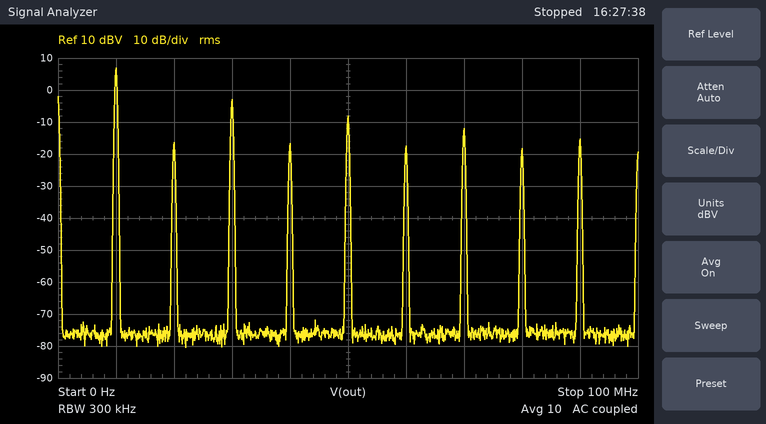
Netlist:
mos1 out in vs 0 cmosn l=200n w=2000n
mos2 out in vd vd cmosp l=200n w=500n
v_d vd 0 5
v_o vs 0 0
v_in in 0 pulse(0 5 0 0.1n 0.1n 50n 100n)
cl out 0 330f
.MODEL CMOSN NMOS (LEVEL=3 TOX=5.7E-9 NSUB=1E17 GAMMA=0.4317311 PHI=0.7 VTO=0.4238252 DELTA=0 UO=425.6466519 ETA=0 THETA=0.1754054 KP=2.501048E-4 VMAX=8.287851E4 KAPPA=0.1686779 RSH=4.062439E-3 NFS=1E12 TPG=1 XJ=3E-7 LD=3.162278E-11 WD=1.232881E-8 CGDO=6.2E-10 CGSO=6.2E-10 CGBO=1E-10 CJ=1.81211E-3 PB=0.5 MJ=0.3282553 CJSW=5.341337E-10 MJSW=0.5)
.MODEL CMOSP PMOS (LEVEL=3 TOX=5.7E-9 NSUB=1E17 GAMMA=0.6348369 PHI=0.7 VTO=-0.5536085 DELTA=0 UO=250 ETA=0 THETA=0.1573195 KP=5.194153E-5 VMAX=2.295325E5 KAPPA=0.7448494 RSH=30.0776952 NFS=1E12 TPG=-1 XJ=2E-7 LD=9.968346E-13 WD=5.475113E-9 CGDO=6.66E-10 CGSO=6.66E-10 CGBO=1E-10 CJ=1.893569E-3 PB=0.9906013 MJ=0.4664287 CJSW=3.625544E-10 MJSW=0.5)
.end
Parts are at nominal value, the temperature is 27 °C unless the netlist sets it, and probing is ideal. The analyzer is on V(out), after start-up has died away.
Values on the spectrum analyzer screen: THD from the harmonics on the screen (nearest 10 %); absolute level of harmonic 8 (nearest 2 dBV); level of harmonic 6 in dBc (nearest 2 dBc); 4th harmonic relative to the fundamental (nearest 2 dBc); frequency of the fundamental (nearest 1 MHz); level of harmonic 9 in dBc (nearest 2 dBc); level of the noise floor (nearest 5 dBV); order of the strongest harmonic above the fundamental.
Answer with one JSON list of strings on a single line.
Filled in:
["40 %", "-18 dBV", "-24 dBc", "-24 dBc", "10 MHz", "-22 dBc", "-75 dBV", "3"]
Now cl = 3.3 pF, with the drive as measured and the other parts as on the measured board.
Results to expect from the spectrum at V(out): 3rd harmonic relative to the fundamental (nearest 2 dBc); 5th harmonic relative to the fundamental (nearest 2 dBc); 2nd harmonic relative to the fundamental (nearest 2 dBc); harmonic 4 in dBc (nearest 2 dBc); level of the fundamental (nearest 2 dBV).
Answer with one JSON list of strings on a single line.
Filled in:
["-12 dBc", "-18 dBc", "-10 dBc", "-16 dBc", "4 dBV"]
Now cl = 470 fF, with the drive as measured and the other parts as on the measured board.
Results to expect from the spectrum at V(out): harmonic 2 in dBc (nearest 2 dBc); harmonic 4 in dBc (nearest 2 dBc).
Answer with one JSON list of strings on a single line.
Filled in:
["-20 dBc", "-22 dBc"]
